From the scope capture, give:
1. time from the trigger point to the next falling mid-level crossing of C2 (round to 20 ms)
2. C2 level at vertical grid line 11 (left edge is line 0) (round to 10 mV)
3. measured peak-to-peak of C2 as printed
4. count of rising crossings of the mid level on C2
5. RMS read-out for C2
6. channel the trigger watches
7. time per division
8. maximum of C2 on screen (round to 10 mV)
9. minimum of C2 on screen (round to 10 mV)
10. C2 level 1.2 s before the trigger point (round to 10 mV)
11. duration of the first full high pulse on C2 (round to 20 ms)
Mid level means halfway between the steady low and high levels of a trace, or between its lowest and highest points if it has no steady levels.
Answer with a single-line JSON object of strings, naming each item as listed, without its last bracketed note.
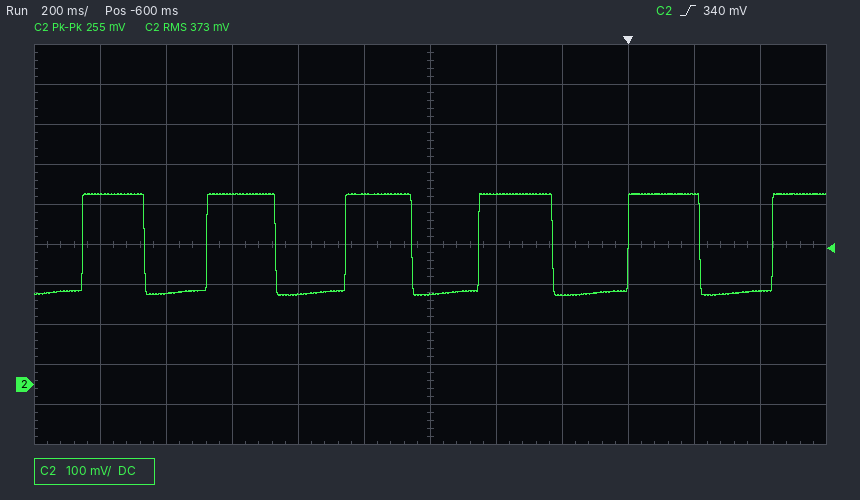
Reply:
{"time from the trigger point to the next falling mid-level crossing of C2": "220 ms", "C2 level at vertical grid line 11 (left edge is line 0)": "230 mV", "measured peak-to-peak of C2 as printed": "255 mV", "count of rising crossings of the mid level on C2": "6", "RMS read-out for C2": "373 mV", "channel the trigger watches": "C2", "time per division": "200 ms", "maximum of C2 on screen": "480 mV", "minimum of C2 on screen": "220 mV", "C2 level 1.2 s before the trigger point": "480 mV", "duration of the first full high pulse on C2": "180 ms"}
